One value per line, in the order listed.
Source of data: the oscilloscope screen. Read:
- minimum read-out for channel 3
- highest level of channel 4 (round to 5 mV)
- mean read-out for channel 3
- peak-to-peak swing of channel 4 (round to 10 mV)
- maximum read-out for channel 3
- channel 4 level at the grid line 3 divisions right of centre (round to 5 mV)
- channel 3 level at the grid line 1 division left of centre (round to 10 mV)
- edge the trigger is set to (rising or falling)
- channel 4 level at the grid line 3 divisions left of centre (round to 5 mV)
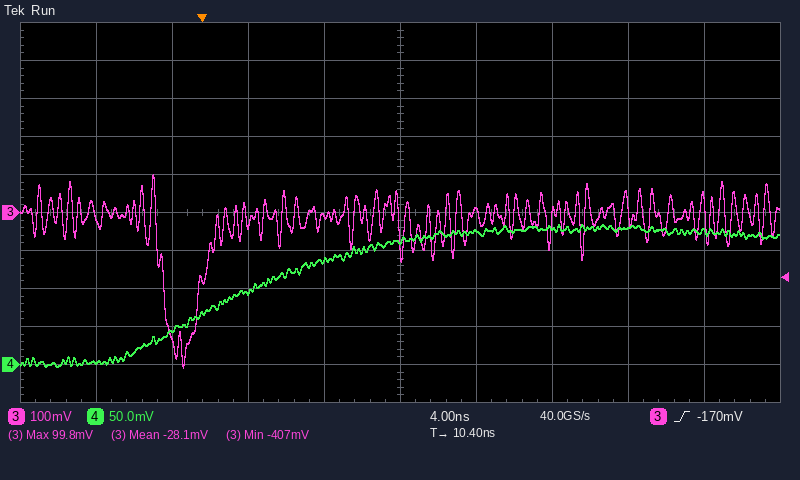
-407 mV
185 mV
-28.1 mV
190 mV
99.8 mV
180 mV
-10 mV
rising
45 mV
